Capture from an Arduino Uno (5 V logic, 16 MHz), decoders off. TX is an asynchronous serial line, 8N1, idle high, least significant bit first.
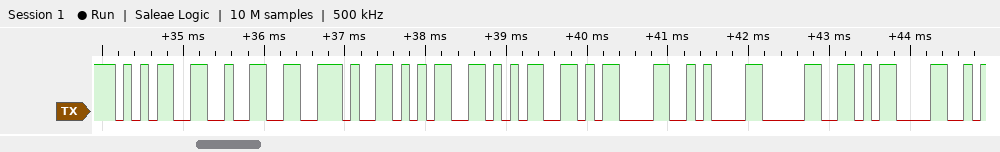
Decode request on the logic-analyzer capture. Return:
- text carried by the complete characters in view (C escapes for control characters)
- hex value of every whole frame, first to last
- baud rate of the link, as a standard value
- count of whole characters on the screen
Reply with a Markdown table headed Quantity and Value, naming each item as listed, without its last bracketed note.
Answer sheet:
| Quantity | Value |
|---|---|
| text carried by the complete characters in view | "52.55\r\n0\r" |
| hex value of every whole frame, first to last | 0x35 0x32 0x2E 0x35 0x35 0x0D 0x0A 0x30 0x0D |
| baud rate of the link, as a standard value | 9600 baud |
| count of whole characters on the screen | 9 |
